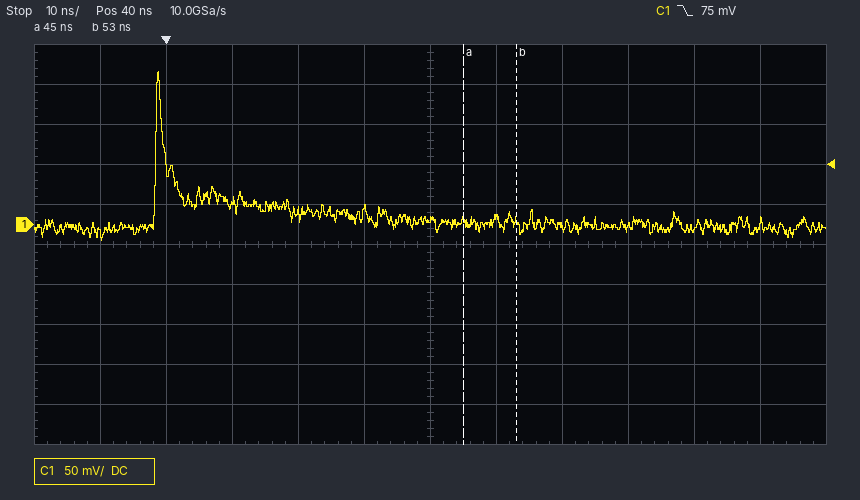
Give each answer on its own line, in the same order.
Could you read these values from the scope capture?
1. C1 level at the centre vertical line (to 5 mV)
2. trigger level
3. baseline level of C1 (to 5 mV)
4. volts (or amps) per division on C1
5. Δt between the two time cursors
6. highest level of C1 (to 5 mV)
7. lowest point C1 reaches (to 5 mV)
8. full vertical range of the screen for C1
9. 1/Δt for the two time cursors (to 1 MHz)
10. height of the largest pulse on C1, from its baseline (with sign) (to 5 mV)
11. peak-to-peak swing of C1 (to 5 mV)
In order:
5 mV
75 mV
0 mV
50 mV
8 ns
190 mV
-20 mV
500 mV
125 MHz
+190 mV
210 mV
